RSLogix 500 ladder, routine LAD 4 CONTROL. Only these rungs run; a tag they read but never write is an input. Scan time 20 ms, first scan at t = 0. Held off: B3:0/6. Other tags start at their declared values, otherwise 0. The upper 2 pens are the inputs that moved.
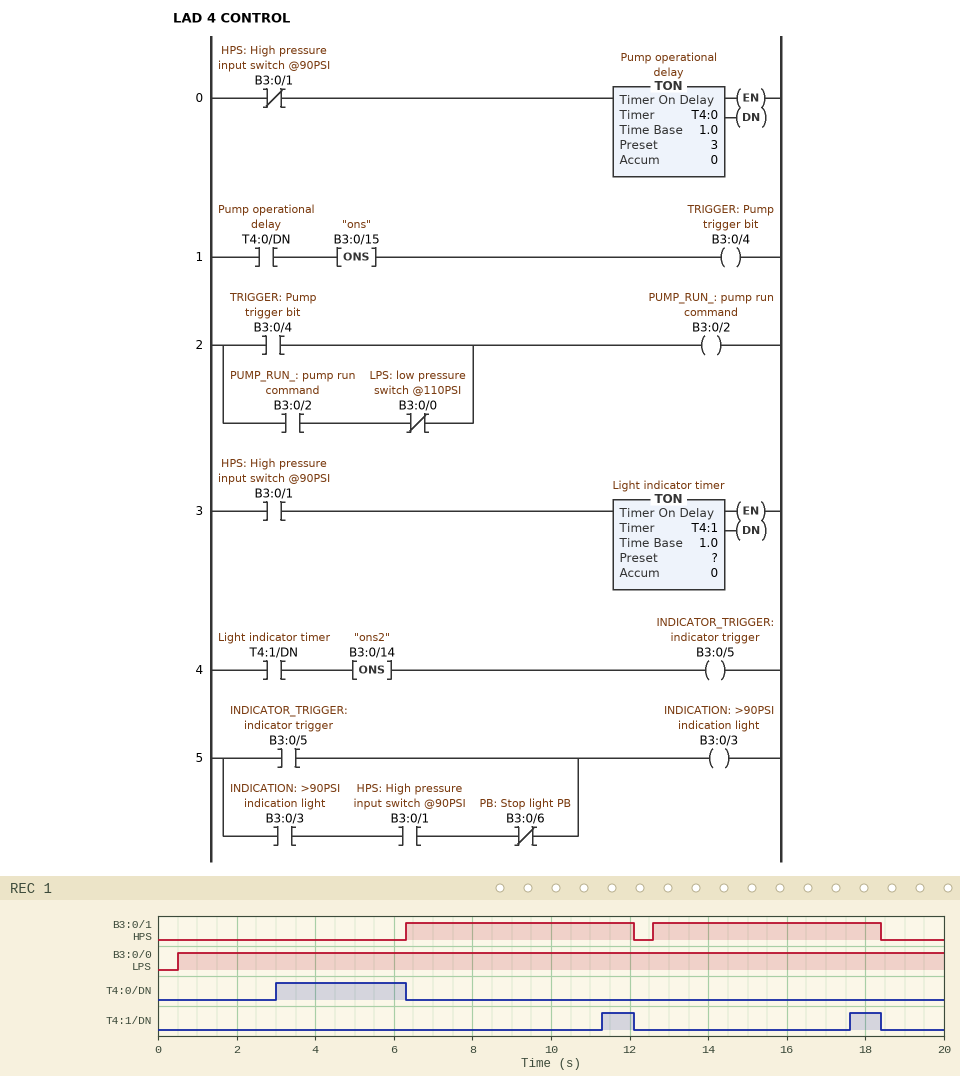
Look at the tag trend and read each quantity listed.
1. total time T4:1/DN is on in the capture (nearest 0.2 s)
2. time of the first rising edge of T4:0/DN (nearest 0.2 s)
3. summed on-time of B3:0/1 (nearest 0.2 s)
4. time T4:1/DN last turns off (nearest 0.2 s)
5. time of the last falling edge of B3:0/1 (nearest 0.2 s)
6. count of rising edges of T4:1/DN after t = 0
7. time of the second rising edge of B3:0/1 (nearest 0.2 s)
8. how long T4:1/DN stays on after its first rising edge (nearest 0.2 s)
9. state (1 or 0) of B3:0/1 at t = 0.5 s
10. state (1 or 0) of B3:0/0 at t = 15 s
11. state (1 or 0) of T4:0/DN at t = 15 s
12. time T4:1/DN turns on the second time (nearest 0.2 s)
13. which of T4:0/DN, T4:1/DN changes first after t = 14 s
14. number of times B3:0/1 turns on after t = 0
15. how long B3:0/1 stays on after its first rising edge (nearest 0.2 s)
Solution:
1.6 s
3.0 s
11.6 s
18.4 s
18.4 s
2
12.6 s
0.8 s
0
1
0
17.6 s
T4:1/DN
2
5.8 s
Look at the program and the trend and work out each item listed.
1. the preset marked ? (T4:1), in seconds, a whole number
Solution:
5 s
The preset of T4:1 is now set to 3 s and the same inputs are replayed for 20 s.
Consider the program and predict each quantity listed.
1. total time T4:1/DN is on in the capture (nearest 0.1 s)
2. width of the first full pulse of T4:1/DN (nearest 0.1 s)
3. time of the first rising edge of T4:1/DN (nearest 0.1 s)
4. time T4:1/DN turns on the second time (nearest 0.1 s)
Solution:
5.6 s
2.8 s
9.3 s
15.6 s
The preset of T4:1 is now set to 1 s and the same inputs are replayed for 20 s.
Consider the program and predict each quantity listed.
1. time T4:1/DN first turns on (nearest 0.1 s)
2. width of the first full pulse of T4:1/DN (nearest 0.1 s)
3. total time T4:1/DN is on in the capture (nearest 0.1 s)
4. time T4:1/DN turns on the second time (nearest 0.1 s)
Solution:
7.3 s
4.8 s
9.6 s
13.6 s
